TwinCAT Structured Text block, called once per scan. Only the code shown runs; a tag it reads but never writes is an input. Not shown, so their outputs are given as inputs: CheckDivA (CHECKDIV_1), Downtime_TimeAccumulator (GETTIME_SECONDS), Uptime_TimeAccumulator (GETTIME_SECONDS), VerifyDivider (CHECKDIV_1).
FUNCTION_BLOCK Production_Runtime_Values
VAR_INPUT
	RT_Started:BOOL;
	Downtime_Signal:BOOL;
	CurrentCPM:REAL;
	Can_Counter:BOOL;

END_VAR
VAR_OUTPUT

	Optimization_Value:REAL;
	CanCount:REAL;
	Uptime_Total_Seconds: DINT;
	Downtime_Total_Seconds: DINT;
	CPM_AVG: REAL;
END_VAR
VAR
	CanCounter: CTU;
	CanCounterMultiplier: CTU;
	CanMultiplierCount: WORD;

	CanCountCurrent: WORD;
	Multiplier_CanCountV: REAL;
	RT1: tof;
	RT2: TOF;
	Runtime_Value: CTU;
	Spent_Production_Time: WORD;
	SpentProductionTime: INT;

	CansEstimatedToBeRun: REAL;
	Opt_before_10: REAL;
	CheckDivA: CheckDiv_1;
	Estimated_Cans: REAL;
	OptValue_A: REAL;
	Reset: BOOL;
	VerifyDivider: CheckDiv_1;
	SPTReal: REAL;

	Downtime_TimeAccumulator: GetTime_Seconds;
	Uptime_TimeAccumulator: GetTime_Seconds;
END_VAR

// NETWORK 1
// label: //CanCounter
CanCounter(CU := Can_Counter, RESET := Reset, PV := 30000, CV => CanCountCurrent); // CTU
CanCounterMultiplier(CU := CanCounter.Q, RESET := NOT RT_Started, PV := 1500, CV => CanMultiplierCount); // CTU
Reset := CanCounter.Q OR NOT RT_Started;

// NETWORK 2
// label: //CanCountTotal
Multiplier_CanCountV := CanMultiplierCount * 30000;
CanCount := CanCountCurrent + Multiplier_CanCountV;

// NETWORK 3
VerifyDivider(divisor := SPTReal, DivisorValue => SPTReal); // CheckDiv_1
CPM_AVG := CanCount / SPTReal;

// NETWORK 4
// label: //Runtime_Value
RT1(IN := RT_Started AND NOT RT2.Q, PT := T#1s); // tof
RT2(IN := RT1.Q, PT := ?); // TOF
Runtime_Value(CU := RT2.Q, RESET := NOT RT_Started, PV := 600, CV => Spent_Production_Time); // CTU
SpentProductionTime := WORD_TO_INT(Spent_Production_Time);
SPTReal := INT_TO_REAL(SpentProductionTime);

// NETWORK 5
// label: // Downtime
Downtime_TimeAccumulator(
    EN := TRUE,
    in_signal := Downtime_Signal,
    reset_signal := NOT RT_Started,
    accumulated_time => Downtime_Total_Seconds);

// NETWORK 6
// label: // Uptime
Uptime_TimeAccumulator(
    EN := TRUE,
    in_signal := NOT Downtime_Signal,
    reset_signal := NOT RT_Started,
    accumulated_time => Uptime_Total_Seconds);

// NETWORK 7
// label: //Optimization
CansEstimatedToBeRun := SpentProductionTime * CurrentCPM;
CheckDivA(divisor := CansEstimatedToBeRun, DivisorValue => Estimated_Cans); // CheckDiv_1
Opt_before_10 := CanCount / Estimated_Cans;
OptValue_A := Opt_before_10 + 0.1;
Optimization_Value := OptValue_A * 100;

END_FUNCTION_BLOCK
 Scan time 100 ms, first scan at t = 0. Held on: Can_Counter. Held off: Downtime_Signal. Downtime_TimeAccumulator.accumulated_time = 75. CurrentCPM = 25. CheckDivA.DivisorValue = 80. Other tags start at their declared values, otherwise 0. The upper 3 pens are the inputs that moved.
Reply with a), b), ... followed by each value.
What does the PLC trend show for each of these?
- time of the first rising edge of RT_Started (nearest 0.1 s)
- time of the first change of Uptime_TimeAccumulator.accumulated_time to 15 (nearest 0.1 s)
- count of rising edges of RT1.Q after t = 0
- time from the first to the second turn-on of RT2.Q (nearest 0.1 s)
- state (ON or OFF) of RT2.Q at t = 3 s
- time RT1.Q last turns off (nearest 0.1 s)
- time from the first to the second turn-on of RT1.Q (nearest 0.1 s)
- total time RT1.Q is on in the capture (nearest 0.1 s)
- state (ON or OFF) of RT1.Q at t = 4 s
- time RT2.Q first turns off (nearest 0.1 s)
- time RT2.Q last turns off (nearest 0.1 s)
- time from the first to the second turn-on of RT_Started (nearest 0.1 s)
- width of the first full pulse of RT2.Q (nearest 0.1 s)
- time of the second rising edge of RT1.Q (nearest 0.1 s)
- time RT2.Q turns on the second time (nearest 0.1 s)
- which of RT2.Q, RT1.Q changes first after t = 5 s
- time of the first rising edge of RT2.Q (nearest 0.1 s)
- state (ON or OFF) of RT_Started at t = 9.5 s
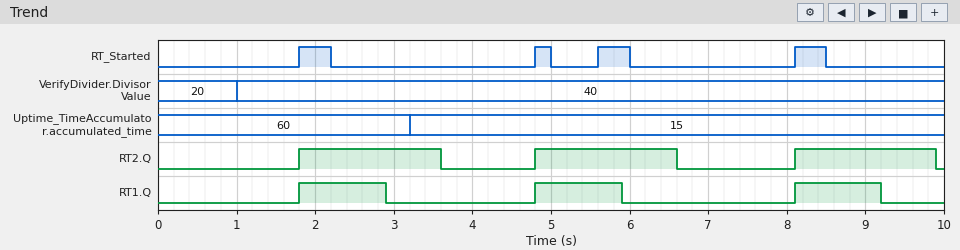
a) 1.8 s
b) 3.2 s
c) 3
d) 3.0 s
e) ON
f) 9.2 s
g) 3.0 s
h) 3.3 s
i) OFF
j) 3.6 s
k) 9.9 s
l) 3.0 s
m) 1.8 s
n) 4.8 s
o) 4.8 s
p) RT1.Q
q) 1.8 s
r) OFF
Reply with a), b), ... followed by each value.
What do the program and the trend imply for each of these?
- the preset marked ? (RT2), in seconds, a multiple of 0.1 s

a) 0.7 s
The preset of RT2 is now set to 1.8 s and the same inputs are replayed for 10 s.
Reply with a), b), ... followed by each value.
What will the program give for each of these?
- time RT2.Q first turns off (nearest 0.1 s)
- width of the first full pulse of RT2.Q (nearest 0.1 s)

a) 4.7 s
b) 2.9 s
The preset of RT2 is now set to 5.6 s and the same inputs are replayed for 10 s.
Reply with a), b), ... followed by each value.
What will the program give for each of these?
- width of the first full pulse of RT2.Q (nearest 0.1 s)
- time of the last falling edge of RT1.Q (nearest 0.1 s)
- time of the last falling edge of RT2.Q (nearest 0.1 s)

a) 6.7 s
b) 2.9 s
c) 8.5 s
